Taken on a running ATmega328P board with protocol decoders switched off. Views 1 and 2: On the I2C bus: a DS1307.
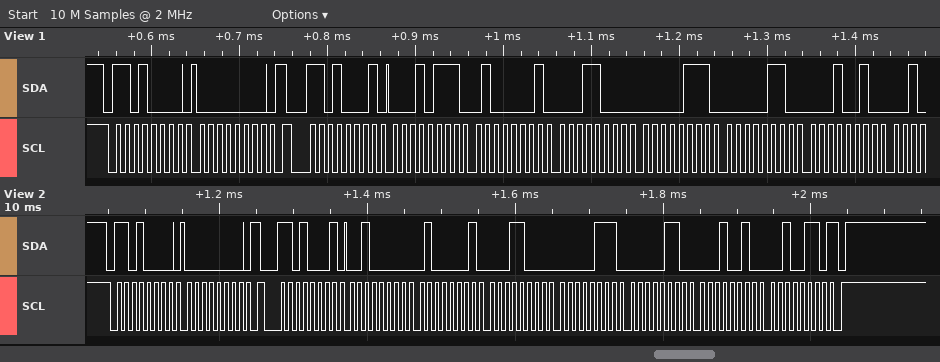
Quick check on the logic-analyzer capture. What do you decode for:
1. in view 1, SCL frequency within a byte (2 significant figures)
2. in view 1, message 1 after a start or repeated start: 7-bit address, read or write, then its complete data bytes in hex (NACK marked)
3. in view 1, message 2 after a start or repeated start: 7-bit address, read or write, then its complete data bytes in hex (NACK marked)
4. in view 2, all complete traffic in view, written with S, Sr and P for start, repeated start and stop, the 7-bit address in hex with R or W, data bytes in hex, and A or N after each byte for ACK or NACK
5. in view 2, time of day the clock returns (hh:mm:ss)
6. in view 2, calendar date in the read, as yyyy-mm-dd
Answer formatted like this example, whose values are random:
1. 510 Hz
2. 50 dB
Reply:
1. 100 kHz
2. 0x68 write: 00
3. 0x68 read: 17 41 18 07 06 12
4. S 68W A 00 A Sr 68R A 20 A 41 A 18 A 07 A 06 A 12 A 26 N P
5. 18:41:20
6. 2026-12-06
